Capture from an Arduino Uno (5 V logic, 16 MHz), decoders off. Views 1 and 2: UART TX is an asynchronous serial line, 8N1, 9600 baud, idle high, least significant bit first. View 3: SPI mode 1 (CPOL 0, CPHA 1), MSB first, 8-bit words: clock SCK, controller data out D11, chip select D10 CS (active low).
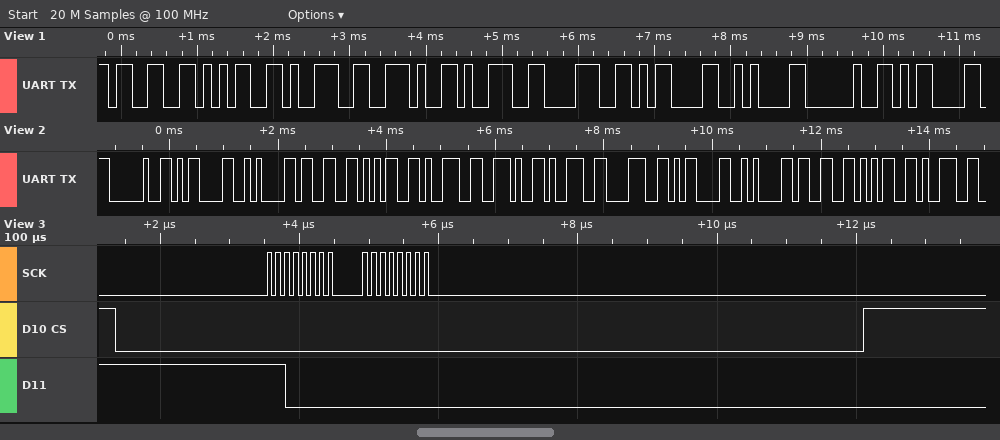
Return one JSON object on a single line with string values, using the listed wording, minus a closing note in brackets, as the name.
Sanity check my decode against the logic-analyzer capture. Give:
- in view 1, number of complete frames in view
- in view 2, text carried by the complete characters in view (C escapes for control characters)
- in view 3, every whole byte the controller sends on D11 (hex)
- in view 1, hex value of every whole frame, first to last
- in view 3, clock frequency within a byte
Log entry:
{"in view 1, number of complete frames in view": "10", "in view 2, text carried by the complete characters in view": "\" \\r\\n359.98\\r\\n359\"", "in view 3, every whole byte the controller sends on D11": "C0 00", "in view 1, hex value of every whole frame, first to last": "33 35 39 2E 39 38 0D 0A 20 0D", "in view 3, clock frequency within a byte": "8 MHz"}
